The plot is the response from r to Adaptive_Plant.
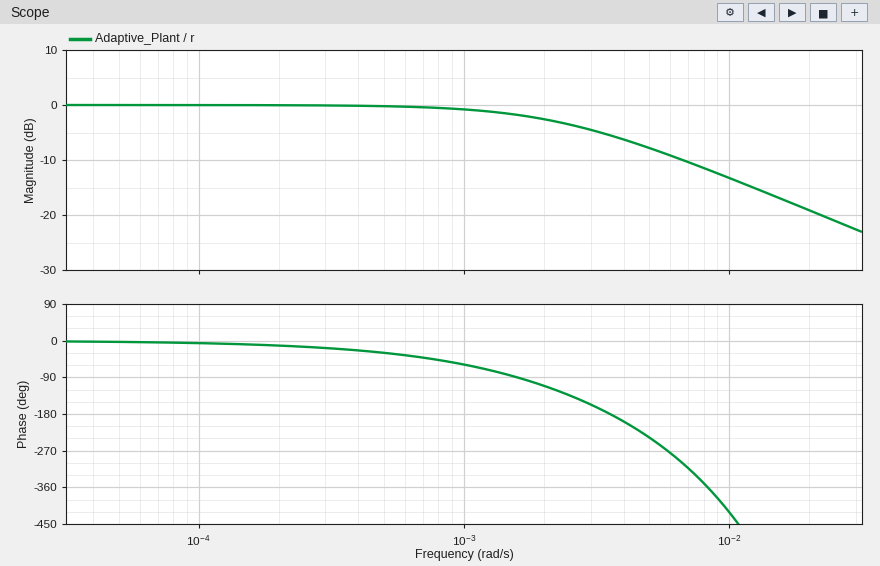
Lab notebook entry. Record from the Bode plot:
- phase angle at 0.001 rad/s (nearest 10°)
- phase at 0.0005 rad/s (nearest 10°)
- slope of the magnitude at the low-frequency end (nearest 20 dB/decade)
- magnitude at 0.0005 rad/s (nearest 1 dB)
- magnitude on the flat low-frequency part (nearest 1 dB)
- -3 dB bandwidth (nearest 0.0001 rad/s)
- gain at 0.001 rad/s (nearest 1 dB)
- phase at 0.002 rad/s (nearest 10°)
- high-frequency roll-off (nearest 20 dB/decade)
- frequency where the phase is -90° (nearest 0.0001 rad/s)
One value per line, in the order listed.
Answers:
-60°
-30°
0 dB/decade
0 dB
0 dB
0.0022 rad/s
-1 dB
-110°
-20 dB/decade
0.0016 rad/s
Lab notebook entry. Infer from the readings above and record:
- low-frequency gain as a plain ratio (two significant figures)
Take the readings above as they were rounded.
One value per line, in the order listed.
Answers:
1.0
